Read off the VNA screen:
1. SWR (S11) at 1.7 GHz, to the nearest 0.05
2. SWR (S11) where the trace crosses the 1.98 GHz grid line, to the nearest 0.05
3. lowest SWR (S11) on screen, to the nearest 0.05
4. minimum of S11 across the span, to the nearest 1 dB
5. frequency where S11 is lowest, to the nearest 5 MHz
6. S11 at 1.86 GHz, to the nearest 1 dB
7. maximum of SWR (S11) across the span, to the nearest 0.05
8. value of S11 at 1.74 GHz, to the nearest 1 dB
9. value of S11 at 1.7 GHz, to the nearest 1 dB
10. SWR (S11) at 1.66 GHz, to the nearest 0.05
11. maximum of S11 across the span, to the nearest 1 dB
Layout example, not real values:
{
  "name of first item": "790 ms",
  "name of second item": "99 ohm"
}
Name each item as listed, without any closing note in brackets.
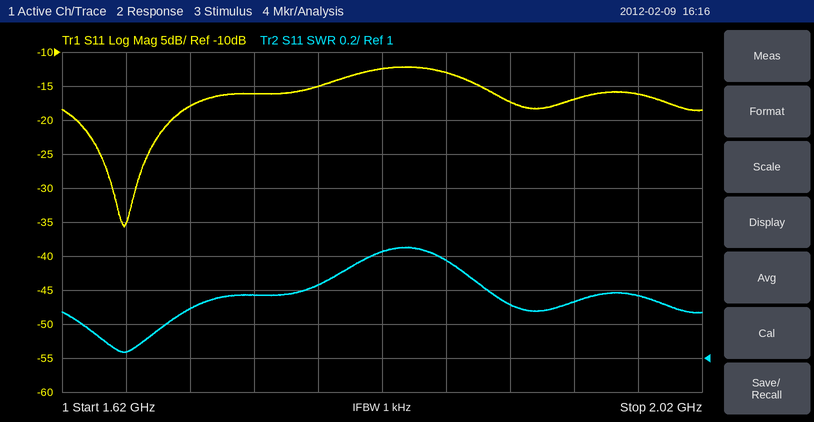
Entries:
{
  "SWR (S11) at 1.7 GHz, to the nearest 0.05": "1.30",
  "SWR (S11) where the trace crosses the 1.98 GHz grid line, to the nearest 0.05": "1.35",
  "lowest SWR (S11) on screen, to the nearest 0.05": "1.05",
  "minimum of S11 across the span, to the nearest 1 dB": "-36 dB",
  "frequency where S11 is lowest, to the nearest 5 MHz": "1.660 GHz",
  "S11 at 1.86 GHz, to the nearest 1 dB": "-13 dB",
  "maximum of SWR (S11) across the span, to the nearest 0.05": "1.65",
  "value of S11 at 1.74 GHz, to the nearest 1 dB": "-16 dB",
  "value of S11 at 1.7 GHz, to the nearest 1 dB": "-18 dB",
  "SWR (S11) at 1.66 GHz, to the nearest 0.05": "1.05",
  "maximum of S11 across the span, to the nearest 1 dB": "-12 dB"
}
